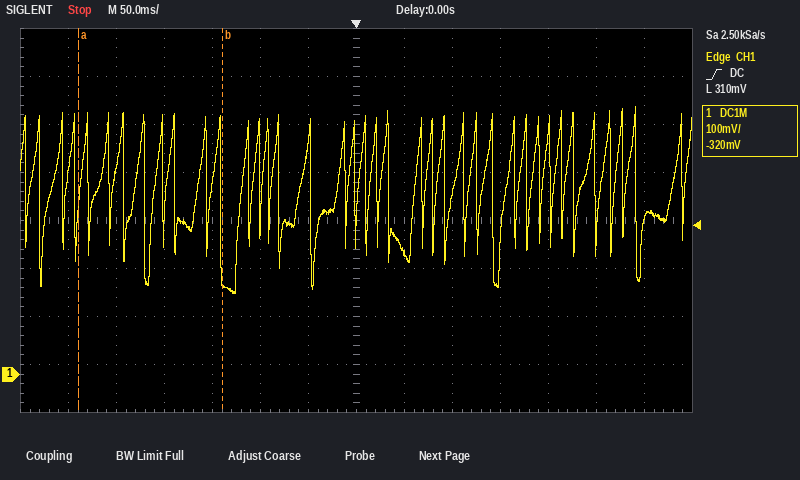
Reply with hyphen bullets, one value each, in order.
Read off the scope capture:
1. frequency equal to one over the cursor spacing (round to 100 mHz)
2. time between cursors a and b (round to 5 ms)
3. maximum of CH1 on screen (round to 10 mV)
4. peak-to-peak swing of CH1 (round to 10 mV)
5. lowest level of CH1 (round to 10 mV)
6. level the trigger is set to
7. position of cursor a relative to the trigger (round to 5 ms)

- 6.7 Hz
- 150 ms
- 560 mV
- 390 mV
- 170 mV
- 310 mV
- -290 ms
